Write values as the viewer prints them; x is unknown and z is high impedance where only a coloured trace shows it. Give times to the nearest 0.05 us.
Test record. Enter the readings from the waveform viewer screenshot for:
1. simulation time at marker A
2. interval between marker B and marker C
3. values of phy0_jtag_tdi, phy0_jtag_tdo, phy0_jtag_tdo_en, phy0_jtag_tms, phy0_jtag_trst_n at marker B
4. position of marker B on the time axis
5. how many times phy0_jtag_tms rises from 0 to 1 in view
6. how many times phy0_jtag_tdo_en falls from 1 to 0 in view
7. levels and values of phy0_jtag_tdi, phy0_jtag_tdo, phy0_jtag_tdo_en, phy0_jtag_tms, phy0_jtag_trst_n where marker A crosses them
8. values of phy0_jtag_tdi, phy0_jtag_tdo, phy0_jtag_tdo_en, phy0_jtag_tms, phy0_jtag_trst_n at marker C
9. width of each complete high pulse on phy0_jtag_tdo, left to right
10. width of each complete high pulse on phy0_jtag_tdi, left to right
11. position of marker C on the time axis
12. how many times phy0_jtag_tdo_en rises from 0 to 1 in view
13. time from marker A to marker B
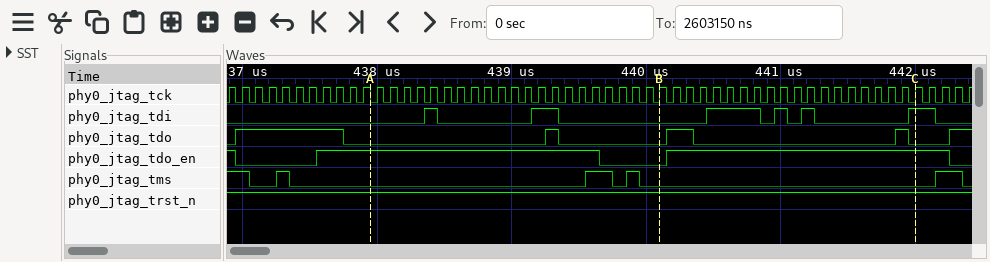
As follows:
437.95 us
1.9 us
phy0_jtag_tdi=0, phy0_jtag_tdo=0, phy0_jtag_tdo_en=0, phy0_jtag_tms=0, phy0_jtag_trst_n=1
440.1 us
4
3
phy0_jtag_tdi=0, phy0_jtag_tdo=0, phy0_jtag_tdo_en=1, phy0_jtag_tms=0, phy0_jtag_trst_n=1
phy0_jtag_tdi=1, phy0_jtag_tdo=0, phy0_jtag_tdo_en=1, phy0_jtag_tms=0, phy0_jtag_trst_n=1
0.8 us, 0.1 us, 0.2 us, 0.1 us
0.1 us, 0.2 us, 0.4 us, 0.1 us, 0.1 us, 0.2 us
442 us
2
2.15 us
